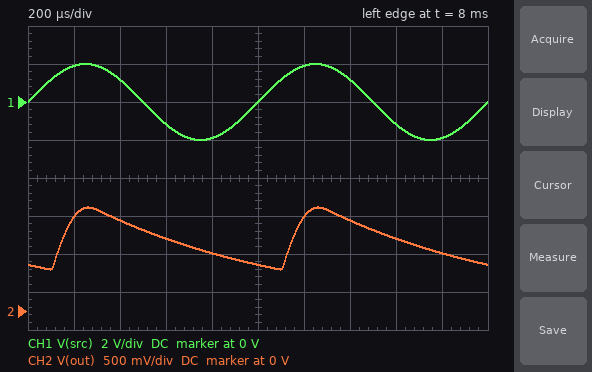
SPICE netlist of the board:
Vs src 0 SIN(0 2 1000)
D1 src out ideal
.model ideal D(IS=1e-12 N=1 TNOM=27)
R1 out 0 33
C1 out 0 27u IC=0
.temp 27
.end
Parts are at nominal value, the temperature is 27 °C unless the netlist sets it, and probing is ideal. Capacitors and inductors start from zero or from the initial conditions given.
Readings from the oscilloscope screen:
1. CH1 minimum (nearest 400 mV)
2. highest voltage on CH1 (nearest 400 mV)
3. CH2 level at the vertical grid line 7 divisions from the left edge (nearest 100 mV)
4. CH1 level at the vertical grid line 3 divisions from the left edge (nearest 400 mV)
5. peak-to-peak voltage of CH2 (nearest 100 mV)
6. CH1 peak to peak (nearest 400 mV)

-2.0 V
2.0 V
1.2 V
-1.2 V
800 mV
4.0 V
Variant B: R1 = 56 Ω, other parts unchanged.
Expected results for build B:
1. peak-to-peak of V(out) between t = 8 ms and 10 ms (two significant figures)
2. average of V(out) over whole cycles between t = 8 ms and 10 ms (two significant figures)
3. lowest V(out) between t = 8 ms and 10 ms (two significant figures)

580 mV
1.1 V
790 mV
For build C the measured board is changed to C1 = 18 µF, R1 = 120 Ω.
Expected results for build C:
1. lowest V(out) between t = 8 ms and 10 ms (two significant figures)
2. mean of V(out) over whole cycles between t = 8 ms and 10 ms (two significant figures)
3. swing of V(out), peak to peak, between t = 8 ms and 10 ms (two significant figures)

930 mV
1.2 V
450 mV
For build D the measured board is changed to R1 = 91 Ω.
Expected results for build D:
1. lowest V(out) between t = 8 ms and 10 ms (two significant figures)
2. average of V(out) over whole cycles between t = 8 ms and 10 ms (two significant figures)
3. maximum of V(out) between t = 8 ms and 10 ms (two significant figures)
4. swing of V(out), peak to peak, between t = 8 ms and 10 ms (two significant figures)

970 mV
1.2 V
1.4 V
410 mV
